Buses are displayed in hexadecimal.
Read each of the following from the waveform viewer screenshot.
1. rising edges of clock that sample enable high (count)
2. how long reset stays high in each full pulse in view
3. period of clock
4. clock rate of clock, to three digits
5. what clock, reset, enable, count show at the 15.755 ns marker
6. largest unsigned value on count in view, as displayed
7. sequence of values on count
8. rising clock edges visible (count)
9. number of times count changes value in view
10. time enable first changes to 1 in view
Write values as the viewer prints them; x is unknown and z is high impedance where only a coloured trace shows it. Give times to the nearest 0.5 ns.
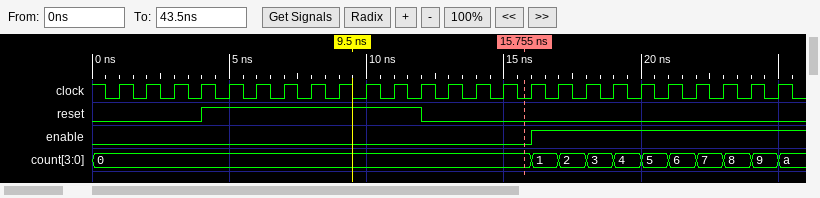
9
8 ns
1 ns
1.00 GHz
clock=0, reset=0, enable=0, count=0
a
0, 1, 2, 3, 4, 5, 6, 7, 8, 9, a
25
10
16 ns
